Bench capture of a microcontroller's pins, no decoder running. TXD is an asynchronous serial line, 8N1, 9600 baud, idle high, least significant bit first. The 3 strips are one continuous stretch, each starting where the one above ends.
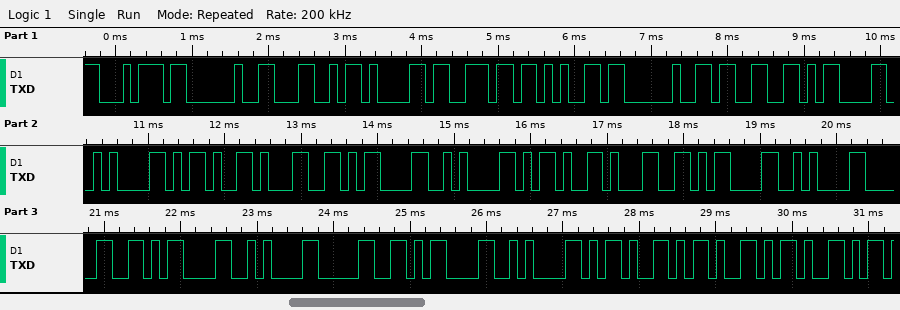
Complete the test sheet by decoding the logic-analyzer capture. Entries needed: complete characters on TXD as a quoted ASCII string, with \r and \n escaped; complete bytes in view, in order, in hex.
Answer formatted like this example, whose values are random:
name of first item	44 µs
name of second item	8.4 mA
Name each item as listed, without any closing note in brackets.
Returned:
complete characters on TXD as a quoted ASCII string, with \r and \n escaped	"t Lane 3\r\n-1\r\n-1\r\n0\r\n0\r\n---"
complete bytes in view, in order, in hex	74 20 4C 61 6E 65 20 33 0D 0A 2D 31 0D 0A 2D 31 0D 0A 30 0D 0A 30 0D 0A 2D 2D 2D
